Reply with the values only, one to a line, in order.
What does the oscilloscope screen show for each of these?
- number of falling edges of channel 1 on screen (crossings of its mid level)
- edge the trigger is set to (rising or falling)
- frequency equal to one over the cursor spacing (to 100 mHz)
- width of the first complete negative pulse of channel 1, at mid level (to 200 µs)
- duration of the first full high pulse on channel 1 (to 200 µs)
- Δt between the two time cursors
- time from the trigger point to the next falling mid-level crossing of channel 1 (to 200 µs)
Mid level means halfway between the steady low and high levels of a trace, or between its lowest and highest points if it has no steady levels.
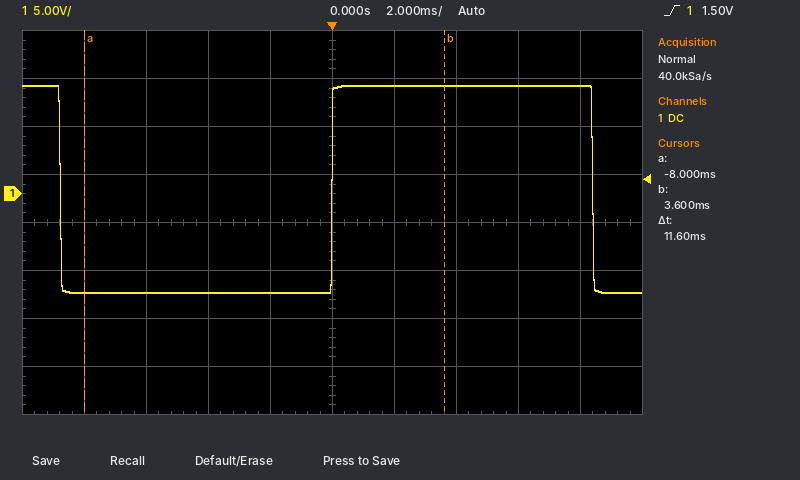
2
rising
86.2 Hz
8.8 ms
8.4 ms
11.6 ms
8.4 ms
